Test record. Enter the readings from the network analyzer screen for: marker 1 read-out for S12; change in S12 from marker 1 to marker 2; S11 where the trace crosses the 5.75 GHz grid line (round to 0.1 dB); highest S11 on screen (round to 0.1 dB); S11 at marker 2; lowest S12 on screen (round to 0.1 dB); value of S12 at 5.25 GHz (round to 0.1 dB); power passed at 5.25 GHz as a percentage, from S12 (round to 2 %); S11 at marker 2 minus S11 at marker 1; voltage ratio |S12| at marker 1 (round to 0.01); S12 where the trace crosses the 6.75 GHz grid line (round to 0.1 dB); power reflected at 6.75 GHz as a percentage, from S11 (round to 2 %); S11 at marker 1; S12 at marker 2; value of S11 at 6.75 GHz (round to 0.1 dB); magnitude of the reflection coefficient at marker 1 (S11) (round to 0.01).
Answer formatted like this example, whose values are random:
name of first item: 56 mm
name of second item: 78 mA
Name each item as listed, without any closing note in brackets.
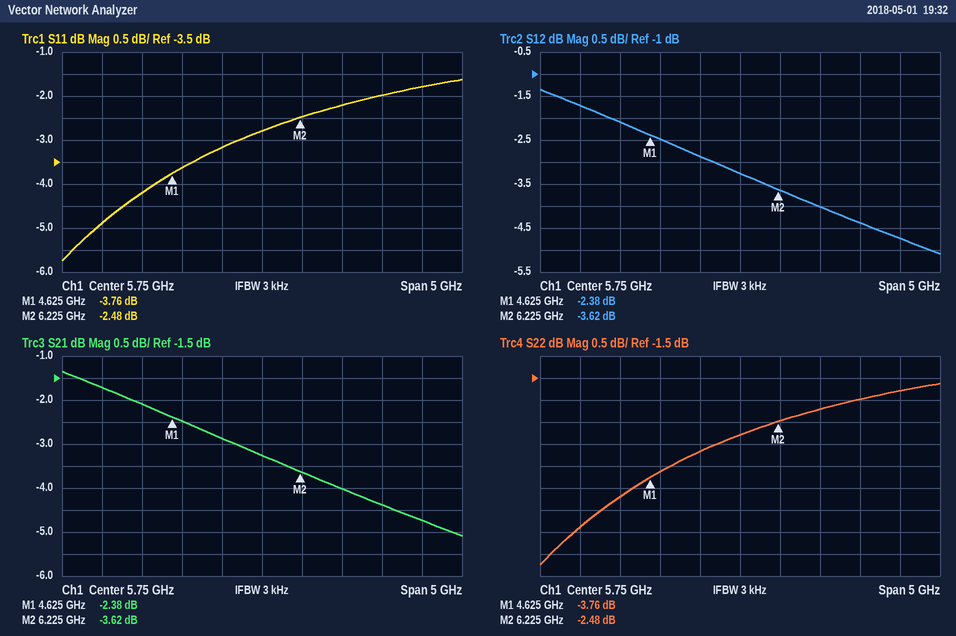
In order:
marker 1 read-out for S12: -2.38 dB
change in S12 from marker 1 to marker 2: -1.24 dB
S11 where the trace crosses the 5.75 GHz grid line: -2.8 dB
highest S11 on screen: -1.6 dB
S11 at marker 2: -2.48 dB
lowest S12 on screen: -5.1 dB
value of S12 at 5.25 GHz: -2.9 dB
power passed at 5.25 GHz as a percentage, from S12: 52 %
S11 at marker 2 minus S11 at marker 1: 1.28 dB
voltage ratio |S12| at marker 1: 0.76
S12 where the trace crosses the 6.75 GHz grid line: -4.0 dB
power reflected at 6.75 GHz as a percentage, from S11: 60 %
S11 at marker 1: -3.76 dB
S12 at marker 2: -3.62 dB
value of S11 at 6.75 GHz: -2.2 dB
magnitude of the reflection coefficient at marker 1 (S11): 0.65
